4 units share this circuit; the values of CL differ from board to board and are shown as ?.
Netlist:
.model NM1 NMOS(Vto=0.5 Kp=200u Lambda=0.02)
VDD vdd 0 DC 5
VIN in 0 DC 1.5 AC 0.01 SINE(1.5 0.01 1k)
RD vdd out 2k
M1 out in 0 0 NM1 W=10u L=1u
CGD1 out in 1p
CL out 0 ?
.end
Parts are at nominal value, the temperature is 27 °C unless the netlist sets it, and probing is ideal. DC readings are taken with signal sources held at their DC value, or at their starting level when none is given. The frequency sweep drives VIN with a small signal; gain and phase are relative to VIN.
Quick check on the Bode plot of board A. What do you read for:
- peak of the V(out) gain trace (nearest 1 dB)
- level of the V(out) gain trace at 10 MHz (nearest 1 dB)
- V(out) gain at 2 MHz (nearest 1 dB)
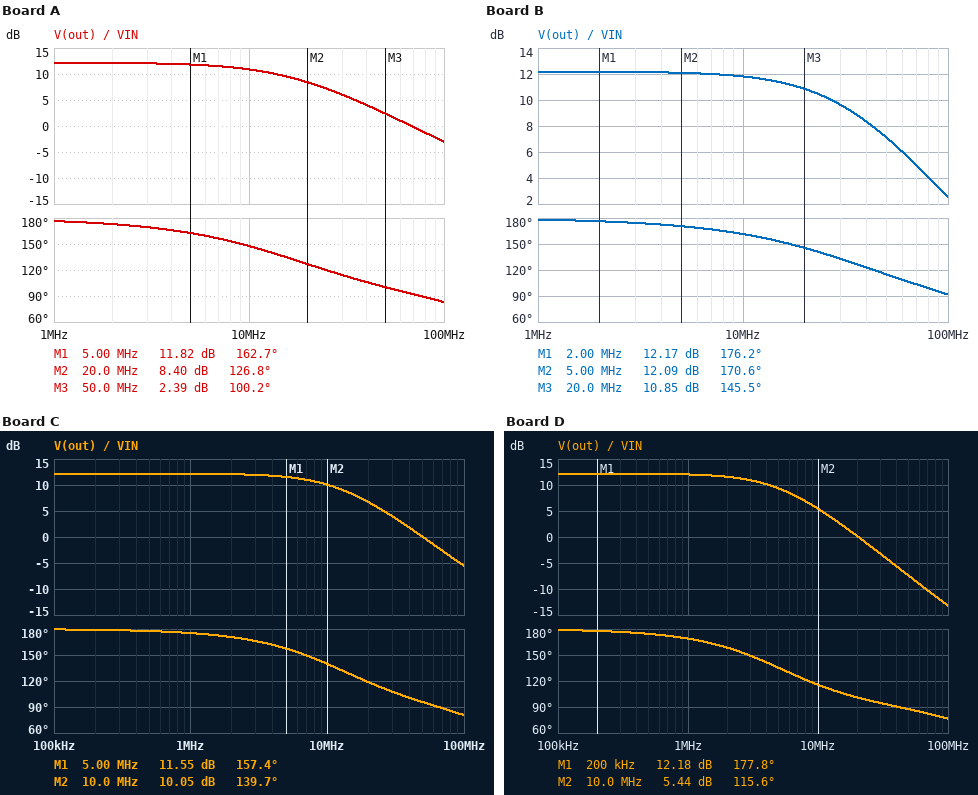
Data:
12 dB
11 dB
12 dB
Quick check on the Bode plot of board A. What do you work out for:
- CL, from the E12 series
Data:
3.9 pF
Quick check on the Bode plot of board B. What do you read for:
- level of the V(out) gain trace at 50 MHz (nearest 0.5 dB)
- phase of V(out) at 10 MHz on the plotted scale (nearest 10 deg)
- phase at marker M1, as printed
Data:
7.0 dB
160 deg
176.2 deg
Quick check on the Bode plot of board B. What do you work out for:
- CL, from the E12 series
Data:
1.5 pF
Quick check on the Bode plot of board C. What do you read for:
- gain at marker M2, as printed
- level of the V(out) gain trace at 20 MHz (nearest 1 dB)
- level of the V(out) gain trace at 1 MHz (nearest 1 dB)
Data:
10.05 dB
7 dB
12 dB
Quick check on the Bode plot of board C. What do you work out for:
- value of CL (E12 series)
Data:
5.6 pF
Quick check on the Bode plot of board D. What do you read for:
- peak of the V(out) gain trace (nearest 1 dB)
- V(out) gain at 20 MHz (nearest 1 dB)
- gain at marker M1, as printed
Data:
12 dB
0 dB
12.18 dB
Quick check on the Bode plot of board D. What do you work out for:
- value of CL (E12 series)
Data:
15 pF
